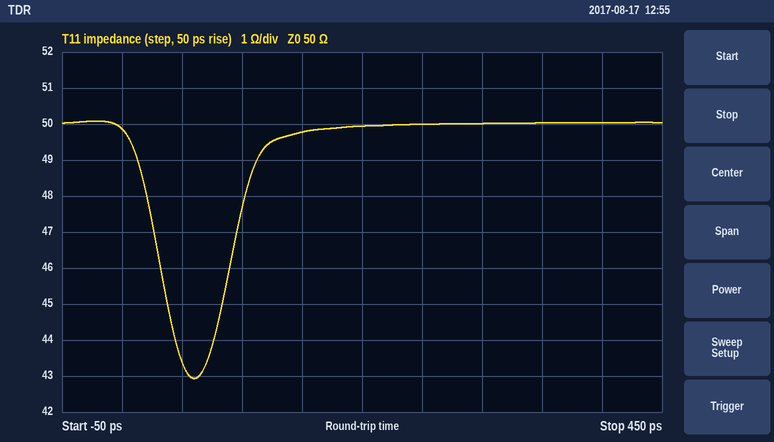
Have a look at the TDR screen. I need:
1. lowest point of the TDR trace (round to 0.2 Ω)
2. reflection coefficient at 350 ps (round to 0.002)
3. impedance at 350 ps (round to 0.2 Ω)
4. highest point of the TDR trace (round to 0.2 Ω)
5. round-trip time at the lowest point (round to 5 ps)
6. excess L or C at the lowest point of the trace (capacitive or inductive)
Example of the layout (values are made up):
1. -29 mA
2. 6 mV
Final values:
1. 43.0 Ω
2. 0.000
3. 50.0 Ω
4. 50.0 Ω
5. 60 ps
6. capacitive
